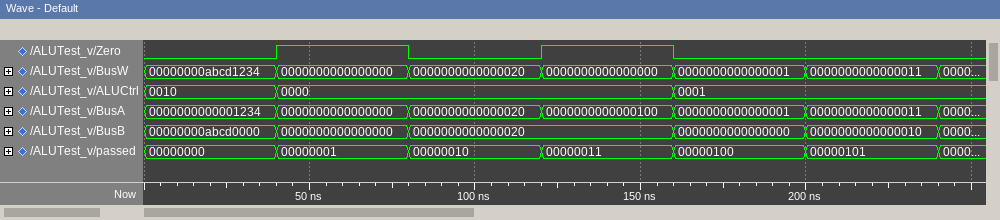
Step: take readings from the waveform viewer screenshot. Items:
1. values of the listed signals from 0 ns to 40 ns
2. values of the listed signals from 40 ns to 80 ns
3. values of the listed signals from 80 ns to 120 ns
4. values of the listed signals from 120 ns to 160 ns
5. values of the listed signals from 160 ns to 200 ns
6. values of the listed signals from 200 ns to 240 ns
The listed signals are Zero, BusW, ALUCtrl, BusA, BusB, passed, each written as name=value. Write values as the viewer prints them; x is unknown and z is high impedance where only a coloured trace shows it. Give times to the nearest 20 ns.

Zero=0, BusW=00000000abcd1234, ALUCtrl=0010, BusA=0000000000001234, BusB=00000000abcd0000, passed=00000000
Zero=1, BusW=0000000000000000, ALUCtrl=0000, BusA=0000000000000000, BusB=0000000000000000, passed=00000001
Zero=0, BusW=0000000000000020, ALUCtrl=0000, BusA=0000000000000020, BusB=0000000000000020, passed=00000010
Zero=1, BusW=0000000000000000, ALUCtrl=0000, BusA=0000000000000100, BusB=0000000000000020, passed=00000011
Zero=0, BusW=0000000000000001, ALUCtrl=0001, BusA=0000000000000001, BusB=0000000000000000, passed=00000100
Zero=0, BusW=0000000000000011, ALUCtrl=0001, BusA=0000000000000011, BusB=0000000000000010, passed=00000101
